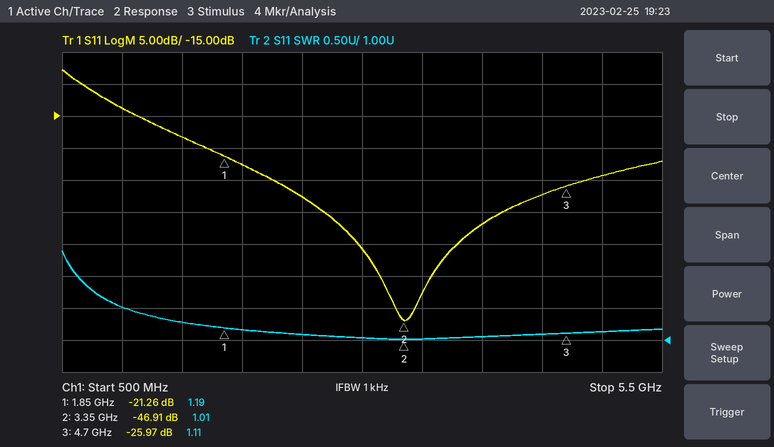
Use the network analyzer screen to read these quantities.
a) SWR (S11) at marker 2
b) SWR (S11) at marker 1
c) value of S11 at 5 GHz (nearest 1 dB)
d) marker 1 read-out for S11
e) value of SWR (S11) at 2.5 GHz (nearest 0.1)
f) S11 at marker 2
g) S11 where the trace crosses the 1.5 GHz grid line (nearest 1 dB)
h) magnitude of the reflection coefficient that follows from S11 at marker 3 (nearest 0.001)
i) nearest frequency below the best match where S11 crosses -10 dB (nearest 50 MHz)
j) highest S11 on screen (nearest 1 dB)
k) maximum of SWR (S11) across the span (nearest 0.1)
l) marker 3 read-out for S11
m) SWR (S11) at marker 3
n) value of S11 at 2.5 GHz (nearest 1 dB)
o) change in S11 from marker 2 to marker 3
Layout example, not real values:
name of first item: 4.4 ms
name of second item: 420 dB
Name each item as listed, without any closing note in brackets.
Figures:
SWR (S11) at marker 2: 1.01
SWR (S11) at marker 1: 1.19
value of S11 at 5 GHz: -24 dB
marker 1 read-out for S11: -21.26 dB
value of SWR (S11) at 2.5 GHz: 1.1
S11 at marker 2: -46.91 dB
S11 where the trace crosses the 1.5 GHz grid line: -18 dB
magnitude of the reflection coefficient that follows from S11 at marker 3: 0.050
nearest frequency below the best match where S11 crosses -10 dB: 650 MHz
highest S11 on screen: -8 dB
maximum of SWR (S11) across the span: 2.4
marker 3 read-out for S11: -25.97 dB
SWR (S11) at marker 3: 1.11
value of S11 at 2.5 GHz: -28 dB
change in S11 from marker 2 to marker 3: 20.94 dB
